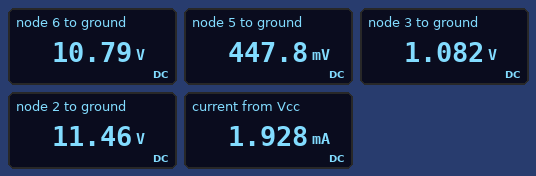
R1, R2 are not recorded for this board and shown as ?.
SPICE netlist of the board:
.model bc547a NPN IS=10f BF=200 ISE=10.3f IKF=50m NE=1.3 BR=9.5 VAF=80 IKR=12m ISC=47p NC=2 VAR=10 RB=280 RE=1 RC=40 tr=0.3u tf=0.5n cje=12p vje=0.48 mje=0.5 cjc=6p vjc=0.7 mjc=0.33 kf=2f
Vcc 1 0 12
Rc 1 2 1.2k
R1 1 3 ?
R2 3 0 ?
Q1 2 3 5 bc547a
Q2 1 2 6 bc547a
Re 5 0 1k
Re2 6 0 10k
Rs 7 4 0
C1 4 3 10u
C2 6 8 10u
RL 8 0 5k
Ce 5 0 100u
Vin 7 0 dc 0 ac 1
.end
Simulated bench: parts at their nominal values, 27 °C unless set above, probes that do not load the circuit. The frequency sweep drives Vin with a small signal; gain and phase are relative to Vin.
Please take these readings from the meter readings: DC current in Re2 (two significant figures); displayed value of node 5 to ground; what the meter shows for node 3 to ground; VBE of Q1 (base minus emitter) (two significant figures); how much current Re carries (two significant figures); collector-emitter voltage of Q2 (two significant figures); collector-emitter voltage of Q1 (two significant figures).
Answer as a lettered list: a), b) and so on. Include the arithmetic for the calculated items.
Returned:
a) (10.79 V) / 10 kΩ = 1.1 mA
b) 447.8 mV
c) 1.082 V
d) 1.082 V - 447.8 mV = 630 mV
e) (447.8 mV) / 1 kΩ = 450 µA
f) 12 V - 10.79 V = 1.2 V
g) 11.46 V - 447.8 mV = 11 V
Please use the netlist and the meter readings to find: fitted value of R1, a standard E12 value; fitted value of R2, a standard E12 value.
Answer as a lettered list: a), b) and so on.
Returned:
a) 27 kΩ
b) 2.7 kΩ
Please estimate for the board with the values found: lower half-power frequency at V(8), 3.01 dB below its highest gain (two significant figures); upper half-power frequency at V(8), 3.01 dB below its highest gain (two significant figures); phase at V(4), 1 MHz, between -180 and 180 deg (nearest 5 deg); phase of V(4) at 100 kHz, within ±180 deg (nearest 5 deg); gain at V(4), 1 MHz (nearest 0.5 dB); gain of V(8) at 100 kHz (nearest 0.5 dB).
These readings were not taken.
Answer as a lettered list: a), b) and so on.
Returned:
a) 31 Hz
b) 5.1 MHz
c) 0 deg
d) 0 deg
e) 0 dB
f) 25.5 dB
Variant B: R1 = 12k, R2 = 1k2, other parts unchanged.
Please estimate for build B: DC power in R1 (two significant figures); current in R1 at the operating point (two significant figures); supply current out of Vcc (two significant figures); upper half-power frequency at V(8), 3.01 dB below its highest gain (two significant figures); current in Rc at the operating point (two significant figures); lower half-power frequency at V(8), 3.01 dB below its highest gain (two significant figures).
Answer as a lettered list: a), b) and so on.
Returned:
a) 9.9 mW
b) 910 µA
c) 2.4 mA
d) 5.0 MHz
e) 460 µA
f) 36 Hz
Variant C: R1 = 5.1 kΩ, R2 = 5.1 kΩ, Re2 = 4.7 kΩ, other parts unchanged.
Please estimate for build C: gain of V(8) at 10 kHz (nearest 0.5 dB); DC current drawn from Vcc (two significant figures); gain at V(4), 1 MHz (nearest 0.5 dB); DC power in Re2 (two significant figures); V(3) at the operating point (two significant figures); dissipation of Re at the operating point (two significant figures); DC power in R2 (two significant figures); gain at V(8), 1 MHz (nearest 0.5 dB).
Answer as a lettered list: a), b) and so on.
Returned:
a) 41.5 dB
b) 7.4 mA
c) 0 dB
d) 5.7 mW
e) 5.9 V
f) 27 mW
g) 6.8 mW
h) 35.5 dB
